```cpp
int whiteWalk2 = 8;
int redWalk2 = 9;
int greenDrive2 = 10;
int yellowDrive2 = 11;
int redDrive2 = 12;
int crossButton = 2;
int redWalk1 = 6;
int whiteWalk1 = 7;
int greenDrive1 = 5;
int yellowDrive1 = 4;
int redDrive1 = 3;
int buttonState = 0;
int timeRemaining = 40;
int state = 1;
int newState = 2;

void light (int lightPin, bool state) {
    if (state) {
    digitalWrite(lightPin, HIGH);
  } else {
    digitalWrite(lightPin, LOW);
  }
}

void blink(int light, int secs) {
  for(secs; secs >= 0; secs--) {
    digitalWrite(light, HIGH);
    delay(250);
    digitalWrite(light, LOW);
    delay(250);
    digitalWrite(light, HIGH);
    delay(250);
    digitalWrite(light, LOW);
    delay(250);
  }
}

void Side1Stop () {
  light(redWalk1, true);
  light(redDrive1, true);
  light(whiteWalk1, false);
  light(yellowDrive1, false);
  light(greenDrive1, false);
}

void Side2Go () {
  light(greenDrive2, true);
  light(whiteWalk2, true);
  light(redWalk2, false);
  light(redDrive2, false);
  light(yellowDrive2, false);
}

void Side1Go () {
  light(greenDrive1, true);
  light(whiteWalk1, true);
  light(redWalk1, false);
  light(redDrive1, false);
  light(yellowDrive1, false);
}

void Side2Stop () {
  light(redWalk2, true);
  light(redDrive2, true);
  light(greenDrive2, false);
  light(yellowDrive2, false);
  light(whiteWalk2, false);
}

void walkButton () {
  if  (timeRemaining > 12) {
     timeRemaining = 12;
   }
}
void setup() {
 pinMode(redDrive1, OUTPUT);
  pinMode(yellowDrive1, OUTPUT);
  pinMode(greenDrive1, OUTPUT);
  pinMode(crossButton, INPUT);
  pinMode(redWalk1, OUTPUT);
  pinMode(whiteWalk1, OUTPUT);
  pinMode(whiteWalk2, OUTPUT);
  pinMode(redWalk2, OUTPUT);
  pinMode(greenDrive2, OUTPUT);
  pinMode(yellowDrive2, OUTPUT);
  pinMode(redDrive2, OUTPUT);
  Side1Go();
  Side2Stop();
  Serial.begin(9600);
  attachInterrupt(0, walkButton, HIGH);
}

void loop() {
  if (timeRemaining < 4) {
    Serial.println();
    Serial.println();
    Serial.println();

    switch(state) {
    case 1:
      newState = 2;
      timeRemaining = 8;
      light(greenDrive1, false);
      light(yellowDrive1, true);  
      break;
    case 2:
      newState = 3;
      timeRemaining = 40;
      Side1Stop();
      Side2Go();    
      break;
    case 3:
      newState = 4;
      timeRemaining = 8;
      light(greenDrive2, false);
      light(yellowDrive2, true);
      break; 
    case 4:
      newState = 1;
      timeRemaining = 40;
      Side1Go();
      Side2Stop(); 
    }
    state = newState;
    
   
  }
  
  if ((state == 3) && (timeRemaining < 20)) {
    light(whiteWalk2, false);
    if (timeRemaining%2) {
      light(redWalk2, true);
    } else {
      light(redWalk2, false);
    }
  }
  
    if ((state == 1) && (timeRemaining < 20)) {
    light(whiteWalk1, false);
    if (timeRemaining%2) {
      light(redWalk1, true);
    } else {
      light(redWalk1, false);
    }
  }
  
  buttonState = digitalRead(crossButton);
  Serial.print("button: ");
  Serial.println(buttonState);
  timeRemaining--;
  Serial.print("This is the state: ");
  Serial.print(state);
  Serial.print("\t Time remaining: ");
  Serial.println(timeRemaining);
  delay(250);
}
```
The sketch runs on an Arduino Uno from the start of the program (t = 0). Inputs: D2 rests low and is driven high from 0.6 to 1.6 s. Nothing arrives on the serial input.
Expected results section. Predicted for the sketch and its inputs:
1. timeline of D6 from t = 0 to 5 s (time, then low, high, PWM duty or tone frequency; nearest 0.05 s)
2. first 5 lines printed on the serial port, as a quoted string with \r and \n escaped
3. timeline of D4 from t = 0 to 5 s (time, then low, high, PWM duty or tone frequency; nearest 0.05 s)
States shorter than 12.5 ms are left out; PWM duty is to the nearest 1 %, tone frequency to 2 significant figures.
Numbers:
0 s low; 1 s high; 1.25 s low; 1.5 s high; 1.75 s low; 2 s high; 2.25 s low; 2.5 s high; 2.75 s low; 4.25 s high
"button: 0\r\nThis is the state: 1\t Time remaining: 39\r\nbutton: 0\r\nThis is the state: 1\t Time remaining: 38\r\nbutton: 0\r\n"
0 s low; 3 s high; 4.25 s low
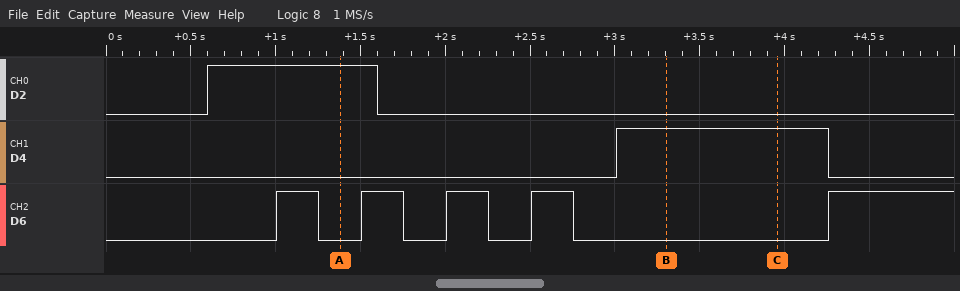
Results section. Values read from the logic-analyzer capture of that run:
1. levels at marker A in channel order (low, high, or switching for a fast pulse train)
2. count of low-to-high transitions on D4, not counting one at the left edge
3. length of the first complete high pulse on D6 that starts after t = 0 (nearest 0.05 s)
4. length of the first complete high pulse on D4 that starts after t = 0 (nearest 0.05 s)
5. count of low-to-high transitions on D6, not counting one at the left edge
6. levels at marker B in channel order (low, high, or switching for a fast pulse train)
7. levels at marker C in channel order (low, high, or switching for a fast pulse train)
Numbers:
D2 high, D4 low, D6 low
1
0.25 s
1.25 s
5
D2 low, D4 high, D6 low
D2 low, D4 high, D6 low
